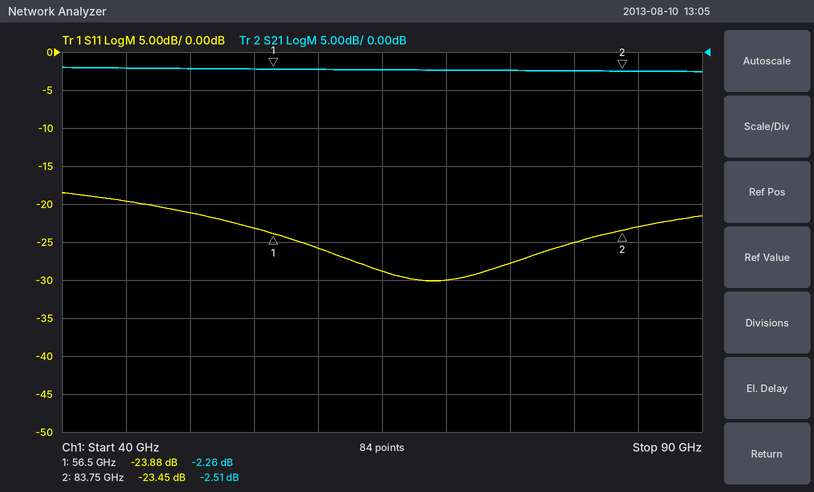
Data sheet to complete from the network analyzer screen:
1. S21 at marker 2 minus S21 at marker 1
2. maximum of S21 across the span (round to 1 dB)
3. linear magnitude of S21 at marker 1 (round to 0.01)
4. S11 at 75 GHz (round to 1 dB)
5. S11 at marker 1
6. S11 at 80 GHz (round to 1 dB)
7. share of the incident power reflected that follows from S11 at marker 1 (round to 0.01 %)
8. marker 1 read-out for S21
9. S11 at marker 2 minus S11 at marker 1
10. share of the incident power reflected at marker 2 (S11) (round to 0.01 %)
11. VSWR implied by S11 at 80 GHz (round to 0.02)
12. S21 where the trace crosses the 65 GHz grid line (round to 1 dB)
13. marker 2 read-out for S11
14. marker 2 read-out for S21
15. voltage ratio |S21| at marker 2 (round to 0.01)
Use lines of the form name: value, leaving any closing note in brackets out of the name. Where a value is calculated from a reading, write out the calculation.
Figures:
S21 at marker 2 minus S21 at marker 1: -2.51 − (-2.26) = -0.25 dB
maximum of S21 across the span: -2 dB
linear magnitude of S21 at marker 1: 10^(-2.26/20) ≈ 0.77
S11 at 75 GHz: -28 dB
S11 at marker 1: -23.88 dB
S11 at 80 GHz: -25 dB
share of the incident power reflected that follows from S11 at marker 1: 10^(-23.88/10) ≈ 0.41 %
marker 1 read-out for S21: -2.26 dB
S11 at marker 2 minus S11 at marker 1: -23.45 − (-23.88) = 0.43 dB
share of the incident power reflected at marker 2 (S11): 10^(-23.45/10) ≈ 0.45 %
VSWR implied by S11 at 80 GHz: |Γ| = 10^(-25/20) = 0.0562; VSWR = (1 + 0.0562)/(1 − 0.0562) ≈ 1.12
S21 where the trace crosses the 65 GHz grid line: -2 dB
marker 2 read-out for S11: -23.45 dB
marker 2 read-out for S21: -2.51 dB
voltage ratio |S21| at marker 2: 10^(-2.51/20) ≈ 0.75
